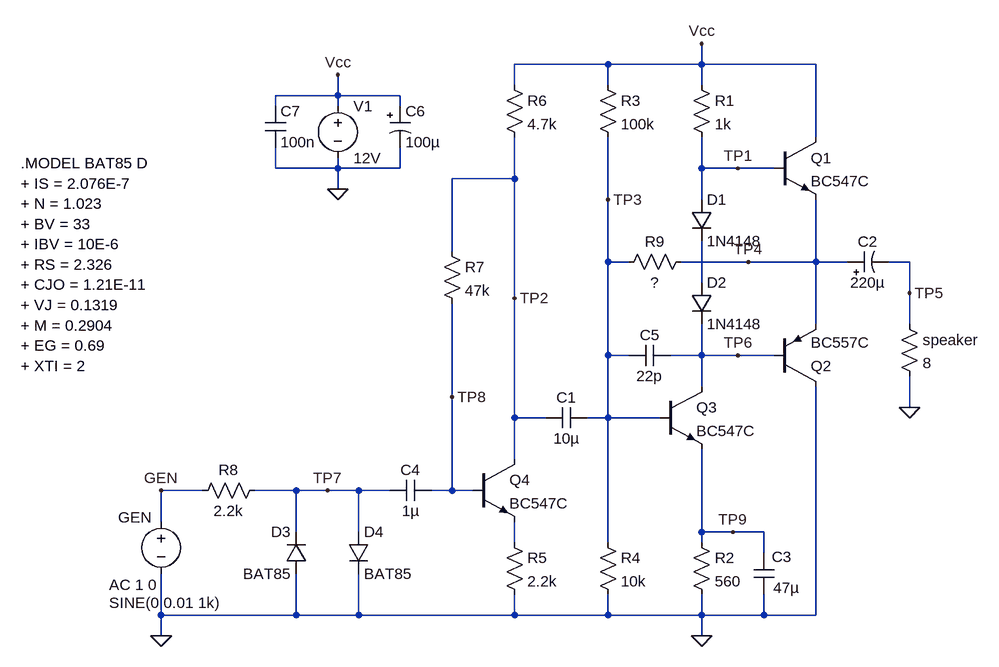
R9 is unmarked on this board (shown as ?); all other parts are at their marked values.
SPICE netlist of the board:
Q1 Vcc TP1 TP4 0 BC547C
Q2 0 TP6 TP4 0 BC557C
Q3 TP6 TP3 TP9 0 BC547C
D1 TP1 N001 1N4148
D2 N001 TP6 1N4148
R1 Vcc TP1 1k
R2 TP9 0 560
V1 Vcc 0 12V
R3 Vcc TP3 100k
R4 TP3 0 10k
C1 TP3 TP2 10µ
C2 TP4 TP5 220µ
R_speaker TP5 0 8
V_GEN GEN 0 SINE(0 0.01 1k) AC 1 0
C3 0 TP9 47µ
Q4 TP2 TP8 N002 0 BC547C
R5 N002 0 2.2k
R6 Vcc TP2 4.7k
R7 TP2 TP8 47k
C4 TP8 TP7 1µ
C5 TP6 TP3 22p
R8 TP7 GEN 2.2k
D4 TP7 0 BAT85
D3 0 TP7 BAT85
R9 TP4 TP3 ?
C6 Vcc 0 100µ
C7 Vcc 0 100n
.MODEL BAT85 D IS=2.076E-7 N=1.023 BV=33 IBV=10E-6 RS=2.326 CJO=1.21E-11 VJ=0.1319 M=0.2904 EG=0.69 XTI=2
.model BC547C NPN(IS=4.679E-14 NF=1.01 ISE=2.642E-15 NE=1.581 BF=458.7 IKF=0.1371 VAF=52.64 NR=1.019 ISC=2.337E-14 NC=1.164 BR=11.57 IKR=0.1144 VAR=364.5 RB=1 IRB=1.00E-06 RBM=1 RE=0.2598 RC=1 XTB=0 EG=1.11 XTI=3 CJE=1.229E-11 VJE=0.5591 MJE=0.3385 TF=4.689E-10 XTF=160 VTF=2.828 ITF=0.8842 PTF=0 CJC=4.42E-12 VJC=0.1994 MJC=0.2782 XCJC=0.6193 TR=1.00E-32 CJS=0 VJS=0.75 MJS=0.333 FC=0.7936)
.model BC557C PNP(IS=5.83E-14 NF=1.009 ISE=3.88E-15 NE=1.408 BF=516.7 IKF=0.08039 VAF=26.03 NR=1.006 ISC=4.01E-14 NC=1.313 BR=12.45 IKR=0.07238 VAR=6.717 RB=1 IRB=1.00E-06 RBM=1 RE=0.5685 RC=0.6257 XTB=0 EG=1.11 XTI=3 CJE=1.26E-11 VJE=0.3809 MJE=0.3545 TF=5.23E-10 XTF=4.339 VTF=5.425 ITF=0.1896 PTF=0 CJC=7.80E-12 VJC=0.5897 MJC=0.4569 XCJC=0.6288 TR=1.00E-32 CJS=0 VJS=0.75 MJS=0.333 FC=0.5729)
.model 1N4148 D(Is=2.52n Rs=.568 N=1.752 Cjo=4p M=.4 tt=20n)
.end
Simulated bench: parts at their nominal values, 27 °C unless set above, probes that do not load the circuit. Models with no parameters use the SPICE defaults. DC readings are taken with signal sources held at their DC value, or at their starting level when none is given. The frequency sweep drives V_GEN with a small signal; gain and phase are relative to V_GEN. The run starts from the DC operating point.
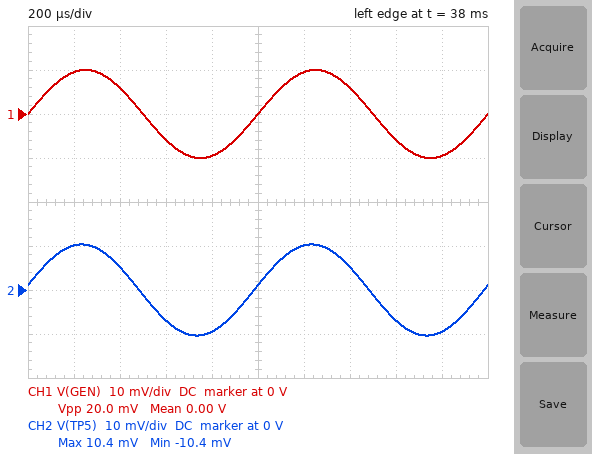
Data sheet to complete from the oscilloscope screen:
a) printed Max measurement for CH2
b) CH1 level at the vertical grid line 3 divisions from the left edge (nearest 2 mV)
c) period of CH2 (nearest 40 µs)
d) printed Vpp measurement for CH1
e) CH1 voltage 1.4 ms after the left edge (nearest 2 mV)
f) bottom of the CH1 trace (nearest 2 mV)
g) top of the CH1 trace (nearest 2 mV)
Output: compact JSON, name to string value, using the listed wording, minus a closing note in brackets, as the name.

{"printed Max measurement for CH2": "10.4 mV", "CH1 level at the vertical grid line 3 divisions from the left edge": "-6 mV", "period of CH2": "1.00 ms", "printed Vpp measurement for CH1": "20.0 mV", "CH1 voltage 1.4 ms after the left edge": "6 mV", "bottom of the CH1 trace": "-10 mV", "top of the CH1 trace": "10 mV"}
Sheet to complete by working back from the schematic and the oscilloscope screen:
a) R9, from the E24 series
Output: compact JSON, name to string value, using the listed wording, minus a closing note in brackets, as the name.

{"R9, from the E24 series": "2.7 kΩ"}
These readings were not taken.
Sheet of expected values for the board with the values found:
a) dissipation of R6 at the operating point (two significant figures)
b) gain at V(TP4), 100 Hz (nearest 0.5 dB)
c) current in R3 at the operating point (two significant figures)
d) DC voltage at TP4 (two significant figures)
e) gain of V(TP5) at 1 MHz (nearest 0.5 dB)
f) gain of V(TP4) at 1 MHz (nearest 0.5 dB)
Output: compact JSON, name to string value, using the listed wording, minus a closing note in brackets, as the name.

{"dissipation of R6 at the operating point": "12 mW", "gain at V(TP4), 100 Hz": "0 dB", "current in R3 at the operating point": "78 µA", "DC voltage at TP4": "5.1 V", "gain of V(TP5) at 1 MHz": "-1.5 dB", "gain of V(TP4) at 1 MHz": "-1.5 dB"}
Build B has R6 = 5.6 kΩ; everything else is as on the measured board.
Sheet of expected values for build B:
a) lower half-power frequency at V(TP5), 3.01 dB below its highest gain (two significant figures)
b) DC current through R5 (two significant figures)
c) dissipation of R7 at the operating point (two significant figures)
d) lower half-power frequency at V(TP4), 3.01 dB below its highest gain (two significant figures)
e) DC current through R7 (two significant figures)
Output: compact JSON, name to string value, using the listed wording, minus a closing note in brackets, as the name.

{"lower half-power frequency at V(TP5), 3.01 dB below its highest gain": "94 Hz", "DC current through R5": "1.4 mA", "dissipation of R7 at the operating point": "470 nW", "lower half-power frequency at V(TP4), 3.01 dB below its highest gain": "9.5 Hz", "DC current through R7": "3.2 µA"}
